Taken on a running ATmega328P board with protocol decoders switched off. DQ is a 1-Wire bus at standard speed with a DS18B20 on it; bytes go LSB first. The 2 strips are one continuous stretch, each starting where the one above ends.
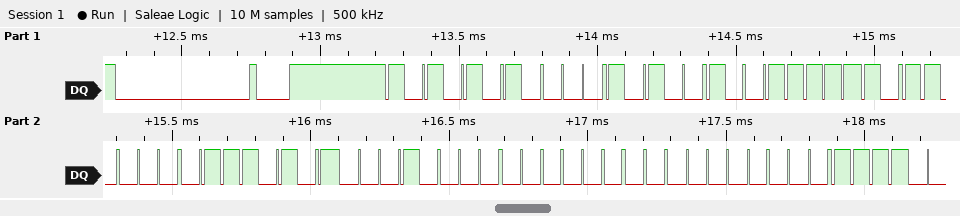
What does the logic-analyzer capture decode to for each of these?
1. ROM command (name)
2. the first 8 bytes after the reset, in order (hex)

Match ROM
55 28 F9 0D AE 08 00 00
